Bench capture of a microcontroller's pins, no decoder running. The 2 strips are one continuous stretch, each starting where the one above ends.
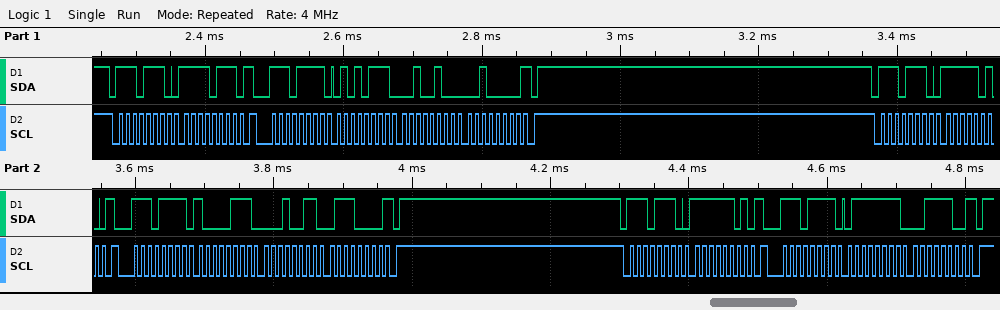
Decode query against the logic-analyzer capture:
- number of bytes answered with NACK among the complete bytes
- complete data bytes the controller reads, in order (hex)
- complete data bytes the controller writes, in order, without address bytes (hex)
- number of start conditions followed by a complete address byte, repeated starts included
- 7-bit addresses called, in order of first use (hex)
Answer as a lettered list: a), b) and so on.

a) 3
b) 57 24 20 87 13 70 7F 3C
c) F7 FA FD
d) 6
e) 0x77
